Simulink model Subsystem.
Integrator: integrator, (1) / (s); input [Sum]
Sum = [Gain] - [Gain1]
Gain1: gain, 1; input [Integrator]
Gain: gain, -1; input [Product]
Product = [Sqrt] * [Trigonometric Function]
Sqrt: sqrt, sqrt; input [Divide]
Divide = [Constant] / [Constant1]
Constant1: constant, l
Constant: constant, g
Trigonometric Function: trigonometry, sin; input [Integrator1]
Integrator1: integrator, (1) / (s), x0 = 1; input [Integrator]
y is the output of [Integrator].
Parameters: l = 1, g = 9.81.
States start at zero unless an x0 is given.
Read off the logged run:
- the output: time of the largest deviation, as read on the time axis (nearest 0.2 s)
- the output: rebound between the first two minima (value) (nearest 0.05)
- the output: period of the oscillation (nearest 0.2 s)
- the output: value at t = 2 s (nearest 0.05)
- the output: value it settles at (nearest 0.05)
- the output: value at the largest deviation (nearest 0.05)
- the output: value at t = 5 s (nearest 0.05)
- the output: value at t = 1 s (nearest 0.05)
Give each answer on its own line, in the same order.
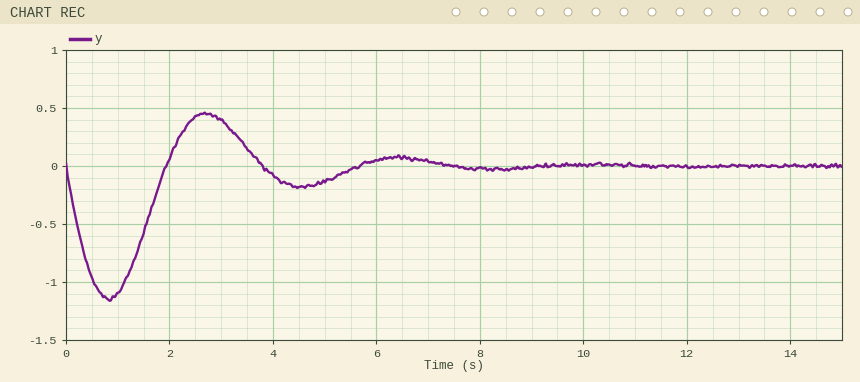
0.8 s
0.45
3.8 s
0.05
0.00
-1.15
-0.15
-1.10
